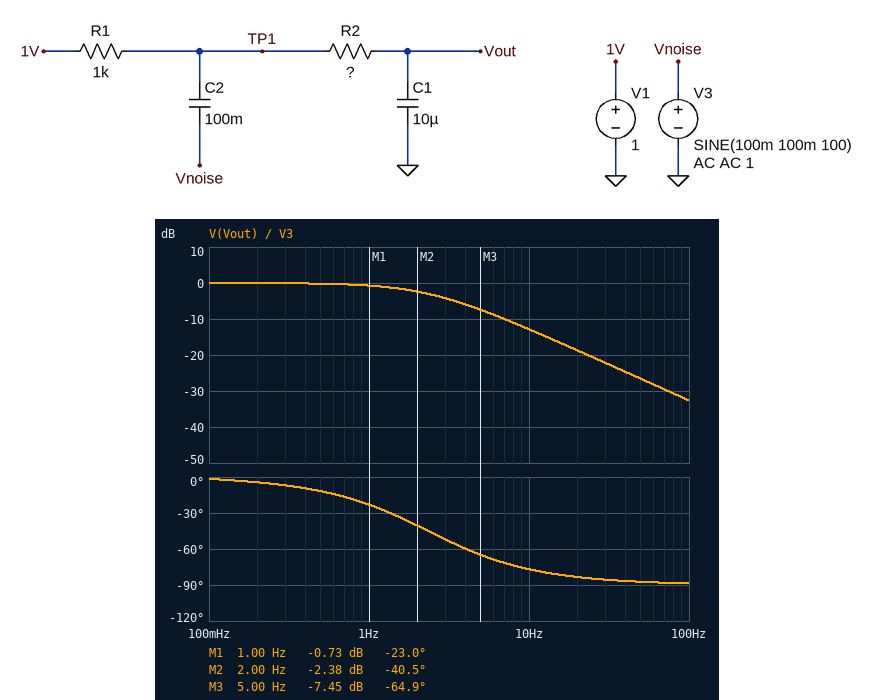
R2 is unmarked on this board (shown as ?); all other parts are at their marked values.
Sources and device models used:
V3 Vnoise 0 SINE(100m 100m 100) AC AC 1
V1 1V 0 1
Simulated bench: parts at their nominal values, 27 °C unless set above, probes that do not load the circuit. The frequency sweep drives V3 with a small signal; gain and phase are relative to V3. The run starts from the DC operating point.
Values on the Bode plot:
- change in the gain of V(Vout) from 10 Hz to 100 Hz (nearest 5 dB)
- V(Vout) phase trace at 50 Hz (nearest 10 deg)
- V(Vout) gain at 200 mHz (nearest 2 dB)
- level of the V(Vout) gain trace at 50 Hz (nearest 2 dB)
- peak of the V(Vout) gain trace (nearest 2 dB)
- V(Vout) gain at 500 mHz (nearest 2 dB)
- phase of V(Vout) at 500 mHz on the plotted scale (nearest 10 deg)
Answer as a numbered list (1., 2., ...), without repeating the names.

1. -20 dB
2. -90 deg
3. 0 dB
4. -26 dB
5. 0 dB
6. 0 dB
7. -10 deg
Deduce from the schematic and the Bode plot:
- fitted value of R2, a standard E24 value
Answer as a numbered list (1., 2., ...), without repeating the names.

1. 6.8 kΩ
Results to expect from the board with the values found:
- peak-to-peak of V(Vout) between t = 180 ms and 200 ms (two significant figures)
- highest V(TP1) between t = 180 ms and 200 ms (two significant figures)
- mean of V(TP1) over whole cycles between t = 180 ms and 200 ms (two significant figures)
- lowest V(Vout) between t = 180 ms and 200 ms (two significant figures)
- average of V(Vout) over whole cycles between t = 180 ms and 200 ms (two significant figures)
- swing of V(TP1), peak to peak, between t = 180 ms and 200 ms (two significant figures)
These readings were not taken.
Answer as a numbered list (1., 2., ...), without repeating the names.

1. 4.7 mV
2. 1.1 V
3. 1.0 V
4. 1.0 V
5. 1.0 V
6. 200 mV
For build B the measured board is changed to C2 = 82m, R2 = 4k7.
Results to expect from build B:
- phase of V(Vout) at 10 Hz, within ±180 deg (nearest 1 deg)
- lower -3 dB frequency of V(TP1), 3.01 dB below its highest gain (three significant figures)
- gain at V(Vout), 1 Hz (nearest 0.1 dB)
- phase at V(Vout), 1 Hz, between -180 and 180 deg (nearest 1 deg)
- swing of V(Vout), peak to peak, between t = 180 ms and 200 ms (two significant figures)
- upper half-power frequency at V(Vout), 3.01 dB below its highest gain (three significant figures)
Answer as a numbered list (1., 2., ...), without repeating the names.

1. -71 deg
2. 1.94 mHz
3. -0.4 dB
4. -16 deg
5. 6.8 mV
6. 3.39 Hz
